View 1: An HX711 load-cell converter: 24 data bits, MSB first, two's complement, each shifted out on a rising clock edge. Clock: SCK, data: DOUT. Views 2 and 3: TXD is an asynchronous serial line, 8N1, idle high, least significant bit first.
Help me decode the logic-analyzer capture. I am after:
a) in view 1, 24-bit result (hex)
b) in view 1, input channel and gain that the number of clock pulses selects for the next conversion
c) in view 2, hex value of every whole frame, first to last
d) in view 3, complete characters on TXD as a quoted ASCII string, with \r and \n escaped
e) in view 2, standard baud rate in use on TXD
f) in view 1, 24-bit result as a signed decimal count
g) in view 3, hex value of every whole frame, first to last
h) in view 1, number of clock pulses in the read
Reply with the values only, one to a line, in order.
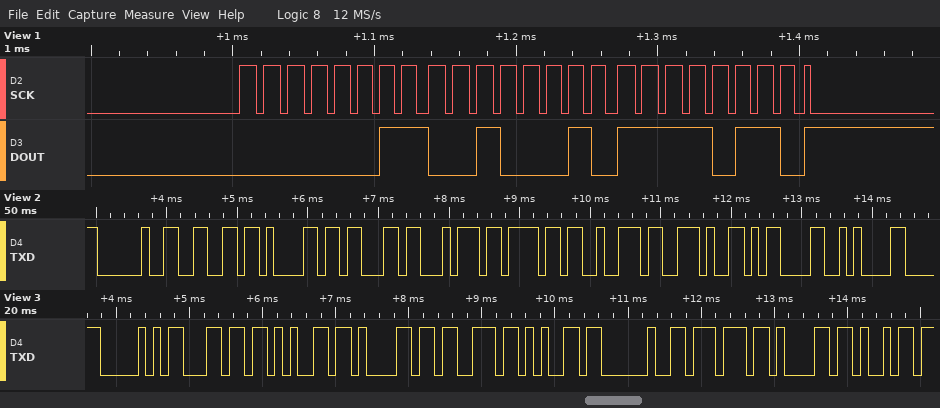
0x0322F6
channel A, gain 128
20 66 61 63 74 6F 72 2E 0D 0A
"Please wai"
9600 baud
205558
0x50 0x6C 0x65 0x61 0x73 0x65 0x20 0x77 0x61 0x69
25
